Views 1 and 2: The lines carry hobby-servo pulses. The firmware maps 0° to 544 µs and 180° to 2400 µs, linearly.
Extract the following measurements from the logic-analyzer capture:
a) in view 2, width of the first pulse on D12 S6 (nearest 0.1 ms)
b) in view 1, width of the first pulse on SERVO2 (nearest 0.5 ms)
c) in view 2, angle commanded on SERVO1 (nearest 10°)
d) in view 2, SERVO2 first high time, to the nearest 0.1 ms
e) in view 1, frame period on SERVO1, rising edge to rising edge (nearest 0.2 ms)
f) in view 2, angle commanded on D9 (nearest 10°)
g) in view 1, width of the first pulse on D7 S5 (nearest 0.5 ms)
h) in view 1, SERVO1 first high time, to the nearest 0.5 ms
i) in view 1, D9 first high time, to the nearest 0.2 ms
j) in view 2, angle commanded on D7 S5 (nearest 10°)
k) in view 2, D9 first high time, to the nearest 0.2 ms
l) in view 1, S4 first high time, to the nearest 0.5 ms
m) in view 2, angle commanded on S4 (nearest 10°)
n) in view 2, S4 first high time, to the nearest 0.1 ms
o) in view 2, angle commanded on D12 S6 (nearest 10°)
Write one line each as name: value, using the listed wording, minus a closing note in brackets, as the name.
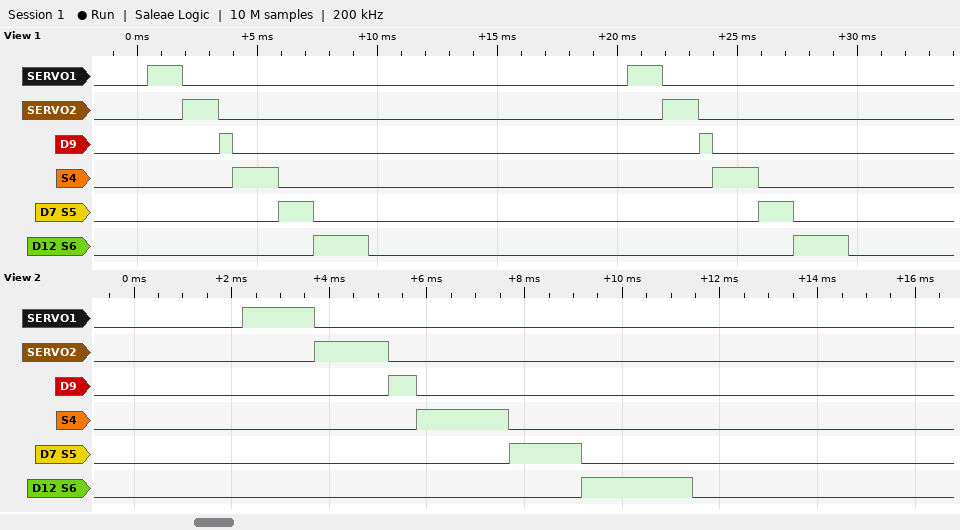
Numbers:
in view 2, width of the first pulse on D12 S6: 2.3 ms
in view 1, width of the first pulse on SERVO2: 1.5 ms
in view 2, angle commanded on SERVO1: 90°
in view 2, SERVO2 first high time, to the nearest 0.1 ms: 1.5 ms
in view 1, frame period on SERVO1, rising edge to rising edge: 20.0 ms
in view 2, angle commanded on D9: 0°
in view 1, width of the first pulse on D7 S5: 1.5 ms
in view 1, SERVO1 first high time, to the nearest 0.5 ms: 1.5 ms
in view 1, D9 first high time, to the nearest 0.2 ms: 0.6 ms
in view 2, angle commanded on D7 S5: 90°
in view 2, D9 first high time, to the nearest 0.2 ms: 0.6 ms
in view 1, S4 first high time, to the nearest 0.5 ms: 2.0 ms
in view 2, angle commanded on S4: 130°
in view 2, S4 first high time, to the nearest 0.1 ms: 1.9 ms
in view 2, angle commanded on D12 S6: 170°
